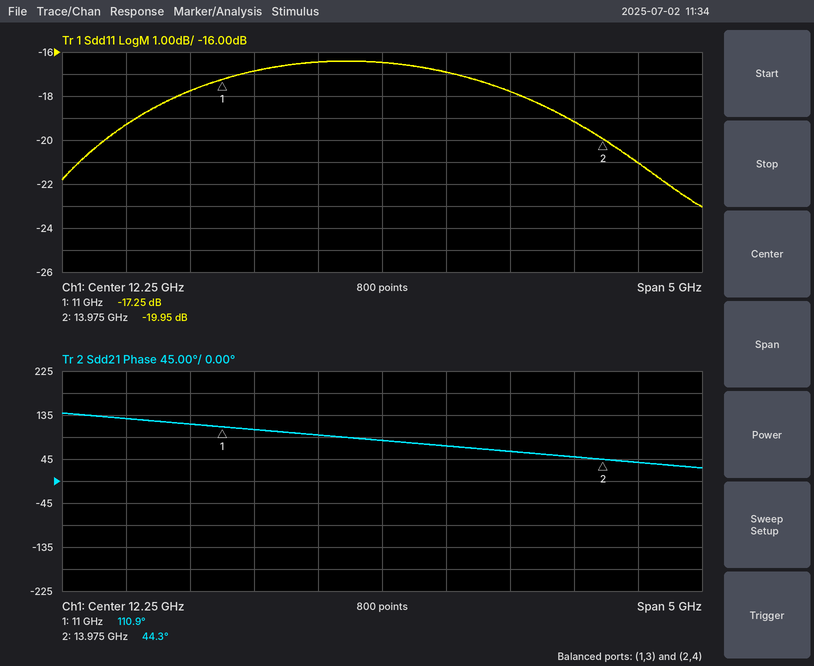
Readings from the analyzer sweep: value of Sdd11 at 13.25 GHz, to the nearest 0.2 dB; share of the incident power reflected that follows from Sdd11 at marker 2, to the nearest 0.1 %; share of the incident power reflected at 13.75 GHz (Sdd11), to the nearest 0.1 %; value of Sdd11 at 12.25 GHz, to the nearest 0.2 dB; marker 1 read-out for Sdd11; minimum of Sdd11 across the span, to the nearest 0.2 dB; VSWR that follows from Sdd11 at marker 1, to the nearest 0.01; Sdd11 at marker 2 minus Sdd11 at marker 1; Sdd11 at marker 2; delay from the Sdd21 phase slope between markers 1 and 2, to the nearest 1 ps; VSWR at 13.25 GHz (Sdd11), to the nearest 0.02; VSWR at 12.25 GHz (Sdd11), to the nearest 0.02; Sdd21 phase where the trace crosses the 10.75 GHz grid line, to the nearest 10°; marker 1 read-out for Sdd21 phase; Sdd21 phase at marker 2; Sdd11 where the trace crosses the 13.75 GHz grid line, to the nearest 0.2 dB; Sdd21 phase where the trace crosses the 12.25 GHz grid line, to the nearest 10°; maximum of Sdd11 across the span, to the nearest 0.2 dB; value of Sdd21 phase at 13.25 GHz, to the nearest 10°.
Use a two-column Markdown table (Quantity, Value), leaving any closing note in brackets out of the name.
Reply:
| Quantity | Value |
|---|---|
| value of Sdd11 at 13.25 GHz, to the nearest 0.2 dB | -17.8 dB |
| share of the incident power reflected that follows from Sdd11 at marker 2, to the nearest 0.1 % | 1.0 % |
| share of the incident power reflected at 13.75 GHz (Sdd11), to the nearest 0.1 % | 1.2 % |
| value of Sdd11 at 12.25 GHz, to the nearest 0.2 dB | -16.4 dB |
| marker 1 read-out for Sdd11 | -17.25 dB |
| minimum of Sdd11 across the span, to the nearest 0.2 dB | -23.0 dB |
| VSWR that follows from Sdd11 at marker 1, to the nearest 0.01 | 1.32 |
| Sdd11 at marker 2 minus Sdd11 at marker 1 | -2.70 dB |
| Sdd11 at marker 2 | -19.95 dB |
| delay from the Sdd21 phase slope between markers 1 and 2, to the nearest 1 ps | 62 ps |
| VSWR at 13.25 GHz (Sdd11), to the nearest 0.02 | 1.30 |
| VSWR at 12.25 GHz (Sdd11), to the nearest 0.02 | 1.36 |
| Sdd21 phase where the trace crosses the 10.75 GHz grid line, to the nearest 10° | 120° |
| marker 1 read-out for Sdd21 phase | 110.9° |
| Sdd21 phase at marker 2 | 44.3° |
| Sdd11 where the trace crosses the 13.75 GHz grid line, to the nearest 0.2 dB | -19.2 dB |
| Sdd21 phase where the trace crosses the 12.25 GHz grid line, to the nearest 10° | 80° |
| maximum of Sdd11 across the span, to the nearest 0.2 dB | -16.4 dB |
| value of Sdd21 phase at 13.25 GHz, to the nearest 10° | 60° |
